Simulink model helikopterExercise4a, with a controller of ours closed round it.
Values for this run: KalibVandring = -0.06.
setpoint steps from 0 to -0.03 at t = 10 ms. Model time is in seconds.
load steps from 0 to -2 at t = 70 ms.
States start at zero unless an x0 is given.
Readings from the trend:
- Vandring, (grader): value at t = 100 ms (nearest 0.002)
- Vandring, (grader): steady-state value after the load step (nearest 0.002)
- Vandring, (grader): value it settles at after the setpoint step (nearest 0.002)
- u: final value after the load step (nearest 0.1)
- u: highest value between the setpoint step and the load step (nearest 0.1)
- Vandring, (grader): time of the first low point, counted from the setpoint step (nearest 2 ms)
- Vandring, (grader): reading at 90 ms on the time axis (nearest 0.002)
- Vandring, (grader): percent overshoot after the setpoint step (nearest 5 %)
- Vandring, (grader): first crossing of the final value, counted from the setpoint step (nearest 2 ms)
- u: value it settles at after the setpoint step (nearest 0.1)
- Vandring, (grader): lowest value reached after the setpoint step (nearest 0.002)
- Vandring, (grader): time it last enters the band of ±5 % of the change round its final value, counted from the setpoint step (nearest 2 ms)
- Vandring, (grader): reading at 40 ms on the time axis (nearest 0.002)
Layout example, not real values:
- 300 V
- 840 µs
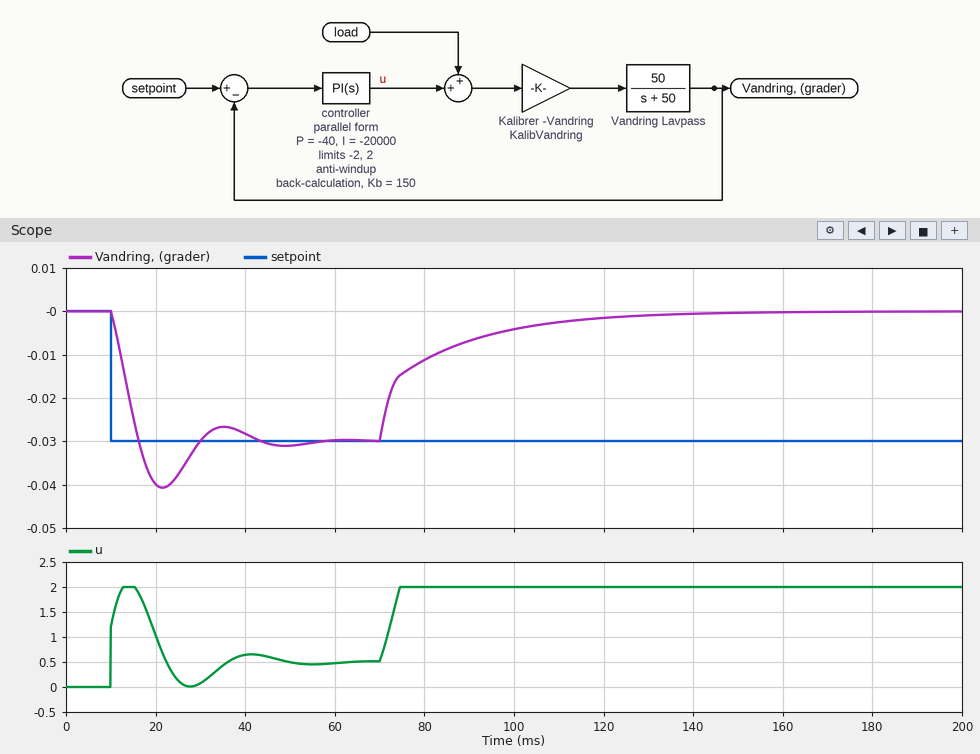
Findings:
- -0.004
- 0.000
- -0.030
- 2.0
- 2.0
- 12 ms
- -0.006
- 35 %
- 6 ms
- 0.5
- -0.040
- 30 ms
- -0.028
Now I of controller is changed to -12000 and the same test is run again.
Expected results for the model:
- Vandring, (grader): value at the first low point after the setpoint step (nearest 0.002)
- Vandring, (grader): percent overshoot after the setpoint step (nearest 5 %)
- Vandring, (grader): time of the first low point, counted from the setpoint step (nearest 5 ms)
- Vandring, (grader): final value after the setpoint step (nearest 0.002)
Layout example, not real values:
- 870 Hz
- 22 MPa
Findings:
- -0.038
- 25 %
- 15 ms
- -0.030
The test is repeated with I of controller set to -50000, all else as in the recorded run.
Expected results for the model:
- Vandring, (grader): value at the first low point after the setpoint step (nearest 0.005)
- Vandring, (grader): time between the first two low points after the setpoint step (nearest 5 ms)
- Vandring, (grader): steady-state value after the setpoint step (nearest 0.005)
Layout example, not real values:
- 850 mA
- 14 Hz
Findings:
- -0.045
- 15 ms
- -0.030
